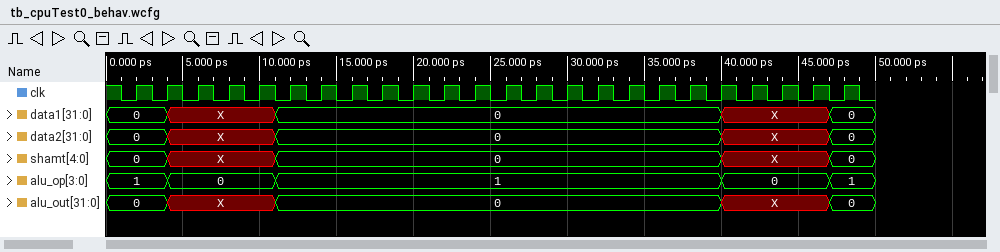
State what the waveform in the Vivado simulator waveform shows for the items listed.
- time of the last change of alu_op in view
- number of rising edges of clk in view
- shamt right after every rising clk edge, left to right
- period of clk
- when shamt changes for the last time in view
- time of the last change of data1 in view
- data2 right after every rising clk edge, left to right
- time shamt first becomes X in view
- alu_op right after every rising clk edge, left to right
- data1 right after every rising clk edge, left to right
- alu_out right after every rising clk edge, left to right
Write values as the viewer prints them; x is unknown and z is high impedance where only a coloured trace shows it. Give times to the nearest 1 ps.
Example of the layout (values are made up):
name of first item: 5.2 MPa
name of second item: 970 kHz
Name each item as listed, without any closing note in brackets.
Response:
time of the last change of alu_op in view: 47 ps
number of rising edges of clk in view: 24
shamt right after every rising clk edge, left to right: 0, X, X, X, X, 0, 0, 0, 0, 0, 0, 0, 0, 0, 0, 0, 0, 0, 0, X, X, X, X, 0
period of clk: 2 ps
when shamt changes for the last time in view: 47 ps
time of the last change of data1 in view: 47 ps
data2 right after every rising clk edge, left to right: 0, X, X, X, X, 0, 0, 0, 0, 0, 0, 0, 0, 0, 0, 0, 0, 0, 0, X, X, X, X, 0
time shamt first becomes X in view: 4 ps
alu_op right after every rising clk edge, left to right: 1, 0, 0, 0, 0, 1, 1, 1, 1, 1, 1, 1, 1, 1, 1, 1, 1, 1, 1, 0, 0, 0, 0, 1
data1 right after every rising clk edge, left to right: 0, X, X, X, X, 0, 0, 0, 0, 0, 0, 0, 0, 0, 0, 0, 0, 0, 0, X, X, X, X, 0
alu_out right after every rising clk edge, left to right: 0, X, X, X, X, 0, 0, 0, 0, 0, 0, 0, 0, 0, 0, 0, 0, 0, 0, X, X, X, X, 0
